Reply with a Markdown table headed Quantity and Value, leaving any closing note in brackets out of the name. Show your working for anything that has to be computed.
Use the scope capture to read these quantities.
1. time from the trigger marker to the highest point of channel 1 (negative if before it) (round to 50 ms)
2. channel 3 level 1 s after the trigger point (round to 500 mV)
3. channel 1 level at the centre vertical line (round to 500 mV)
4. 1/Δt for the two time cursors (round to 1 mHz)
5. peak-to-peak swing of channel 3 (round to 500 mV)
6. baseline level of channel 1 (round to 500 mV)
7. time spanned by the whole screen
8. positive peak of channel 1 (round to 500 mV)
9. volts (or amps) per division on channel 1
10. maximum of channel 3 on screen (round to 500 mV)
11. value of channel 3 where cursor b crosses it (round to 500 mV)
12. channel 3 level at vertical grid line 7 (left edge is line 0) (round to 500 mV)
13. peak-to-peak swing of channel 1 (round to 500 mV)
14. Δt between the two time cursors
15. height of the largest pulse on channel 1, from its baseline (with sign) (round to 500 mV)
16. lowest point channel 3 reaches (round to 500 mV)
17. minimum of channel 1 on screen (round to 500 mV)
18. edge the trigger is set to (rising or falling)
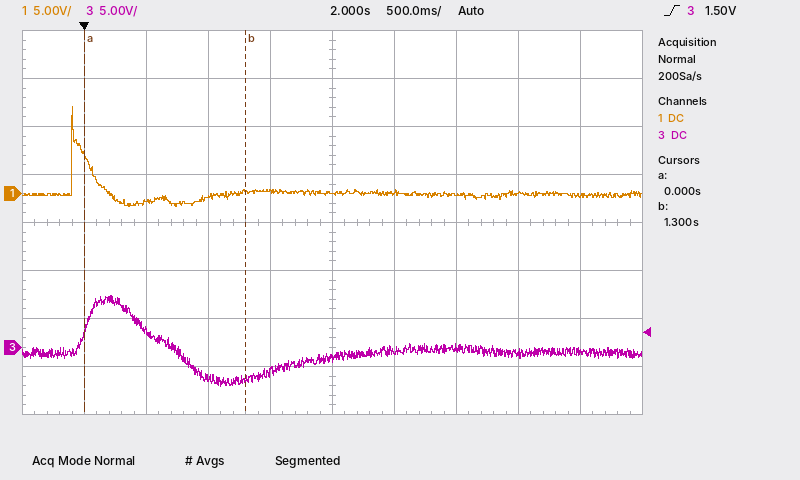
| Quantity | Value |
|---|---|
| time from the trigger marker to the highest point of channel 1 (negative if before it) | -100 ms |
| channel 3 level 1 s after the trigger point | -3.0 V |
| channel 1 level at the centre vertical line | 0.0 V |
| 1/Δt for the two time cursors | 1 / 1.30 s ≈ 769 mHz |
| peak-to-peak swing of channel 3 | 5.5 V − (-4.0 V) = 9.5 V |
| baseline level of channel 1 | 0.0 V |
| time spanned by the whole screen | 5 s |
| positive peak of channel 1 | 9.0 V |
| volts (or amps) per division on channel 1 | 5 V |
| maximum of channel 3 on screen | 5.5 V |
| value of channel 3 where cursor b crosses it | -3.5 V |
| channel 3 level at vertical grid line 7 (left edge is line 0) | 0.0 V |
| peak-to-peak swing of channel 1 | 9.0 V − (-1.5 V) = 10.5 V |
| Δt between the two time cursors | 1.3 s − (0 s) = 1.30 s |
| height of the largest pulse on channel 1, from its baseline (with sign) | 9.0 V − (0.0 V) = +9.0 V |
| lowest point channel 3 reaches | -4.0 V |
| minimum of channel 1 on screen | -1.5 V |
| edge the trigger is set to | rising |
